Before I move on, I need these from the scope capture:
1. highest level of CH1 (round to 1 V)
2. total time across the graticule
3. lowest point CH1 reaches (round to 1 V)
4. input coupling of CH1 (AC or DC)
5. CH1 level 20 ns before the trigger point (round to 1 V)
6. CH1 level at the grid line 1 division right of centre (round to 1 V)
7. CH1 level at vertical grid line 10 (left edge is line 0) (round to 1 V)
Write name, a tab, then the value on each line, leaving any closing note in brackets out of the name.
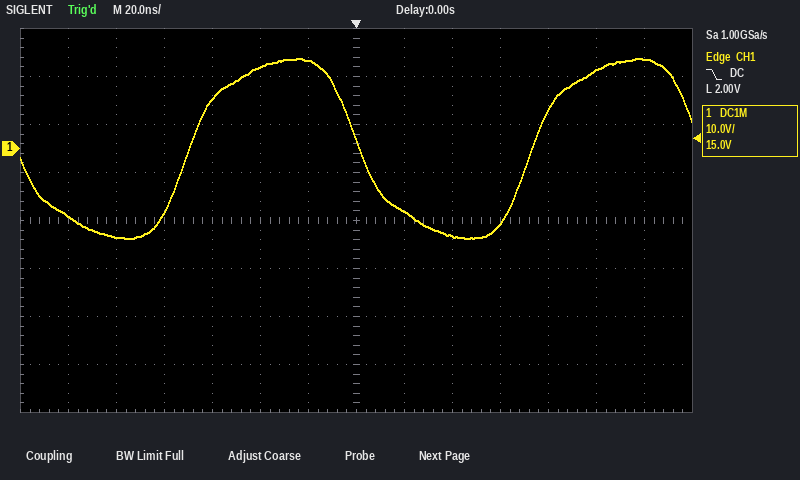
highest level of CH1	19 V
total time across the graticule	280 ns
lowest point CH1 reaches	-19 V
input coupling of CH1	DC
CH1 level 20 ns before the trigger point	18 V
CH1 level at the grid line 1 division right of centre	-13 V
CH1 level at vertical grid line 10 (left edge is line 0)	-16 V
